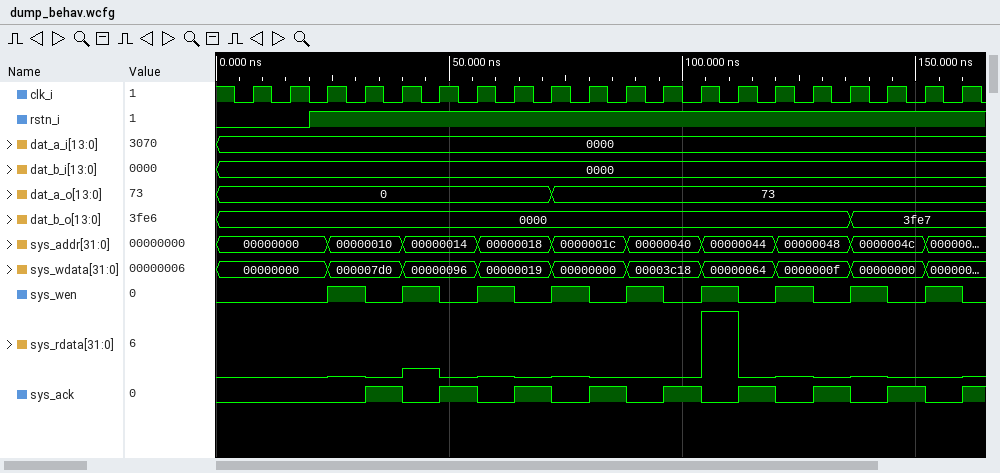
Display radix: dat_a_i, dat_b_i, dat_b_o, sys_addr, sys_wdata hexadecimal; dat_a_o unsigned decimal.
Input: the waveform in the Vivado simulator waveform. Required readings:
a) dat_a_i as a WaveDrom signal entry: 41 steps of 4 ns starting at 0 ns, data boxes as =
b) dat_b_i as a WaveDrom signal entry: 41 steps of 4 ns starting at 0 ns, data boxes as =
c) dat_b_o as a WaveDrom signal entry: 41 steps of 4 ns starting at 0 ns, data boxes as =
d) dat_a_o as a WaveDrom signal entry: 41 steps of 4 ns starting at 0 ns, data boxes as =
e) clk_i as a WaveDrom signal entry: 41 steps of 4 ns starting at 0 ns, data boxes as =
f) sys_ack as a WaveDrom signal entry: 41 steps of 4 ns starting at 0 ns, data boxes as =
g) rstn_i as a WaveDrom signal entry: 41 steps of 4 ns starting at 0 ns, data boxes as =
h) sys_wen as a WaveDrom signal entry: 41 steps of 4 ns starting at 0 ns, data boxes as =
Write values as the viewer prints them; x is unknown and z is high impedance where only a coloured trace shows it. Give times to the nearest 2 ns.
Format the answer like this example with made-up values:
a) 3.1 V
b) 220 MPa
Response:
a) {name: 'dat_a_i', wave: '=........................................', data: '0000'}
b) {name: 'dat_b_i', wave: '=........................................', data: '0000'}
c) {name: 'dat_b_o', wave: '=.................................=......', data: '0000 3fe7'}
d) {name: 'dat_a_o', wave: '=.................=......................', data: '0 73'}
e) {name: 'clk_i', wave: '10101010101010101010101010101010101010101'}
f) {name: 'sys_ack', wave: '0.......1.0.1.0.1.0.1.0.1.0.1.0.1.0.1.0.1'}
g) {name: 'rstn_i', wave: '0....1...................................'}
h) {name: 'sys_wen', wave: '0.....1.0.1.0.1.0.1.0.1.0.1.0.1.0.1.0.1.0'}
